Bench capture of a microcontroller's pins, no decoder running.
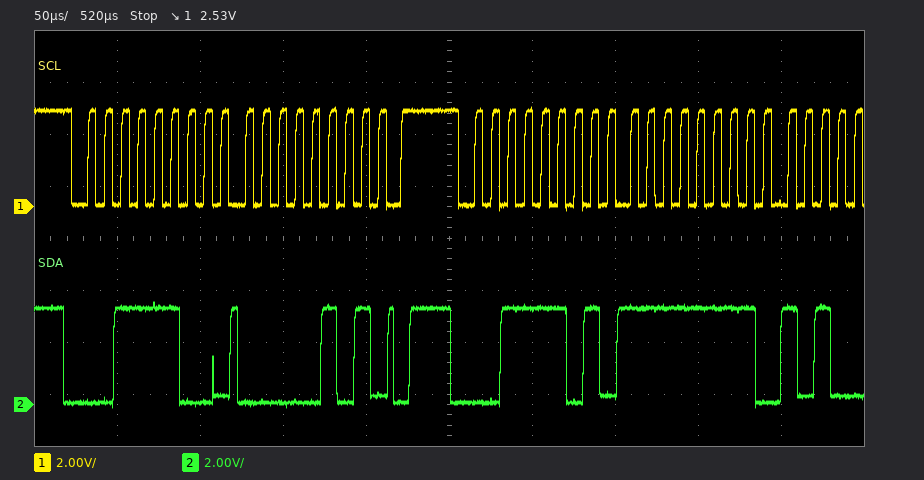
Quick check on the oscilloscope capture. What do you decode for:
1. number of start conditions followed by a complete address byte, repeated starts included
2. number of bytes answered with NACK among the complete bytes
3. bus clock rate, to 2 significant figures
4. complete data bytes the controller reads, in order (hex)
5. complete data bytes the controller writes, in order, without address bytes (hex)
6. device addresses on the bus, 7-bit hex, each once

2
0
100 kHz
FF
05
0x1E
